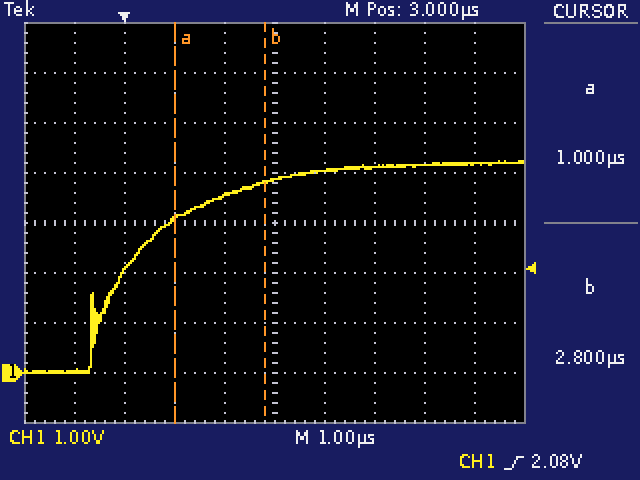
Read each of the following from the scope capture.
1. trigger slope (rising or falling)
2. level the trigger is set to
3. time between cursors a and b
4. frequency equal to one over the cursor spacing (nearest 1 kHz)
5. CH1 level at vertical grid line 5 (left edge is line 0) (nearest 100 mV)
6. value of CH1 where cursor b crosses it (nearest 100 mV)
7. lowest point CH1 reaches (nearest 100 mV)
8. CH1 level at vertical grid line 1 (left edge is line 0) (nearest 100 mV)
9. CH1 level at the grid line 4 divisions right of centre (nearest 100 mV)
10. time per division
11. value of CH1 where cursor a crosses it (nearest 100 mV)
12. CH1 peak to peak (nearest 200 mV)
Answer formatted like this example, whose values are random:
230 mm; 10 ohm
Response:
rising; 2.08 V; 1.8 µs; 556 kHz; 3.9 V; 3.8 V; 0.0 V; 0.0 V; 4.2 V; 1 µs; 3.1 V; 4.2 V
